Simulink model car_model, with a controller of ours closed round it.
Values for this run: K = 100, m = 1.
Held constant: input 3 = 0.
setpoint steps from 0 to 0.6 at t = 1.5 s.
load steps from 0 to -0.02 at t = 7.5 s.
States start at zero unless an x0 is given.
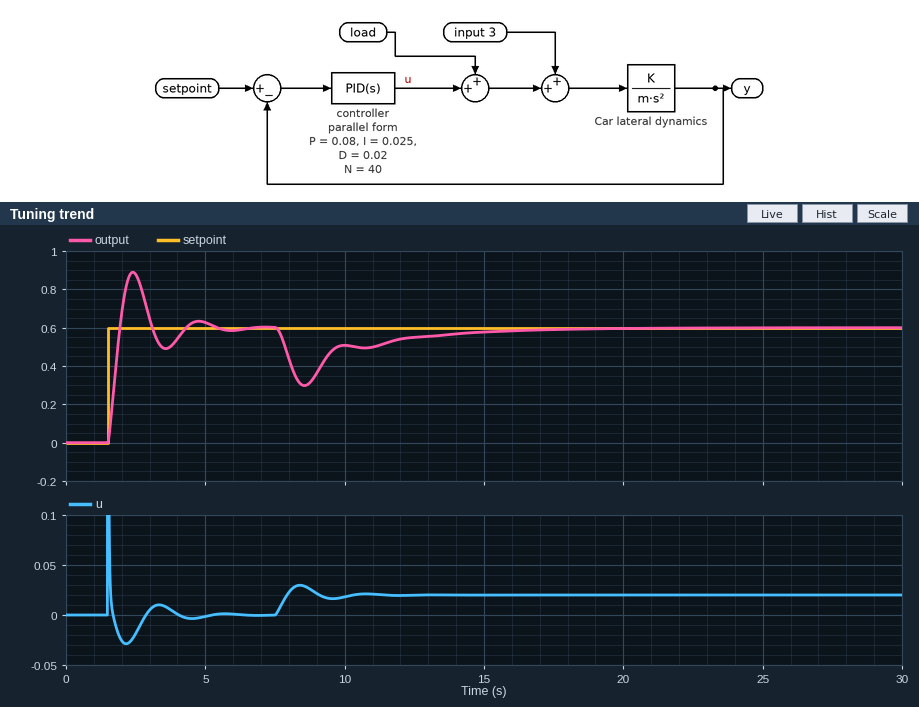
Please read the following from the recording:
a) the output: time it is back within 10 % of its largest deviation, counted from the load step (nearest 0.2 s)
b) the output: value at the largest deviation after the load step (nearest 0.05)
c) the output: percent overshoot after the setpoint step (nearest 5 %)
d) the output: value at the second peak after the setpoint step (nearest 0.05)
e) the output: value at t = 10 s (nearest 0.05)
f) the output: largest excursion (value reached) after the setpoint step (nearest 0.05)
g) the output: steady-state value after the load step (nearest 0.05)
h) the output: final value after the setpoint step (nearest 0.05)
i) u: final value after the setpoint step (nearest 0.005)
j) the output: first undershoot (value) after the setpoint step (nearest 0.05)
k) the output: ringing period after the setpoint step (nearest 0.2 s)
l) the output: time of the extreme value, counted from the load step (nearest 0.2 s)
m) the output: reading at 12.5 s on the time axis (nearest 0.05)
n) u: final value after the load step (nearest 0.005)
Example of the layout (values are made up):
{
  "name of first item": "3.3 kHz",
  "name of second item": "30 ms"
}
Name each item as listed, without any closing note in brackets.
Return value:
{
  "the output: time it is back within 10 % of its largest deviation, counted from the load step": "6.6 s",
  "the output: value at the largest deviation after the load step": "0.30",
  "the output: percent overshoot after the setpoint step": "50 %",
  "the output: value at the second peak after the setpoint step": "0.65",
  "the output: value at t = 10 s": "0.50",
  "the output: largest excursion (value reached) after the setpoint step": "0.90",
  "the output: steady-state value after the load step": "0.60",
  "the output: final value after the setpoint step": "0.60",
  "u: final value after the setpoint step": "0.000",
  "the output: first undershoot (value) after the setpoint step": "0.50",
  "the output: ringing period after the setpoint step": "2.4 s",
  "the output: time of the extreme value, counted from the load step": "1.0 s",
  "the output: reading at 12.5 s on the time axis": "0.55",
  "u: final value after the load step": "0.020"
}
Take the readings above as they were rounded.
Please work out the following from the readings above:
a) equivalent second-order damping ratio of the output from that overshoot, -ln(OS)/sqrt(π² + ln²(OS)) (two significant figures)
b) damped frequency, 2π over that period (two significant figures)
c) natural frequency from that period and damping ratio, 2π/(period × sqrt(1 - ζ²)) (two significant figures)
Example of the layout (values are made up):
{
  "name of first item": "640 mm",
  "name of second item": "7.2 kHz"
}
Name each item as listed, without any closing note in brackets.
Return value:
{
  "equivalent second-order damping ratio of the output from that overshoot, -ln(OS)/sqrt(π² + ln²(OS))": "0.22",
  "damped frequency, 2π over that period": "2.6 rad/s",
  "natural frequency from that period and damping ratio, 2π/(period × sqrt(1 - ζ²))": "2.7 rad/s"
}
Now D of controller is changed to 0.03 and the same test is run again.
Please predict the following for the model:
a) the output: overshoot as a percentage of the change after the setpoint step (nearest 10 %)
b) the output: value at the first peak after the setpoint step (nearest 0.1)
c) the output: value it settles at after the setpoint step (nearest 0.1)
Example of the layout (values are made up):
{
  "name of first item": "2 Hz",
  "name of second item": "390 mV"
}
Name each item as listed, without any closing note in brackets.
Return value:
{
  "the output: overshoot as a percentage of the change after the setpoint step": "30 %",
  "the output: value at the first peak after the setpoint step": "0.8",
  "the output: value it settles at after the setpoint step": "0.6"
}
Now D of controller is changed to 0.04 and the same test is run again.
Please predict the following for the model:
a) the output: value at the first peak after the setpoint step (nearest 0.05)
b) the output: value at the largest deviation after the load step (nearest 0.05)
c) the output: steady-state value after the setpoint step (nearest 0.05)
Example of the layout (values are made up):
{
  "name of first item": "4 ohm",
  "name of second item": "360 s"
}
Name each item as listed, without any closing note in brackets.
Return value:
{
  "the output: value at the first peak after the setpoint step": "0.75",
  "the output: value at the largest deviation after the load step": "0.35",
  "the output: steady-state value after the setpoint step": "0.60"
}
